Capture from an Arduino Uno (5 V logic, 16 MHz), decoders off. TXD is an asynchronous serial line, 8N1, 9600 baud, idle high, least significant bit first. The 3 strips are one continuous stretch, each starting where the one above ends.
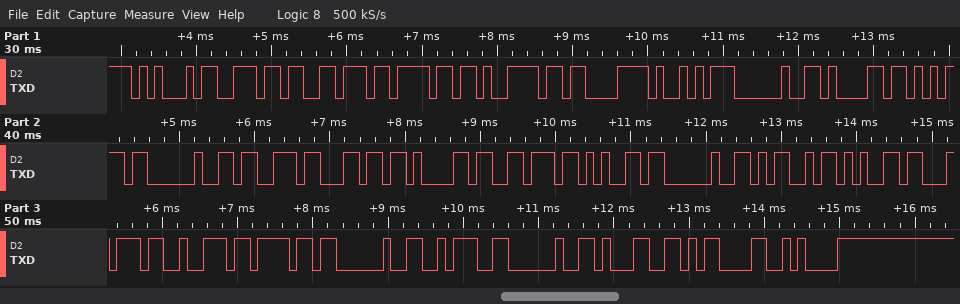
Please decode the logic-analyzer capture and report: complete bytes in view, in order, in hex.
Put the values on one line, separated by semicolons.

45 6E 76 6F 79 C3 A9 20 61 75 20 73 6C 61 76 65 20 4D 65 74 72 6F 20 3A 20 31 0D 0A
